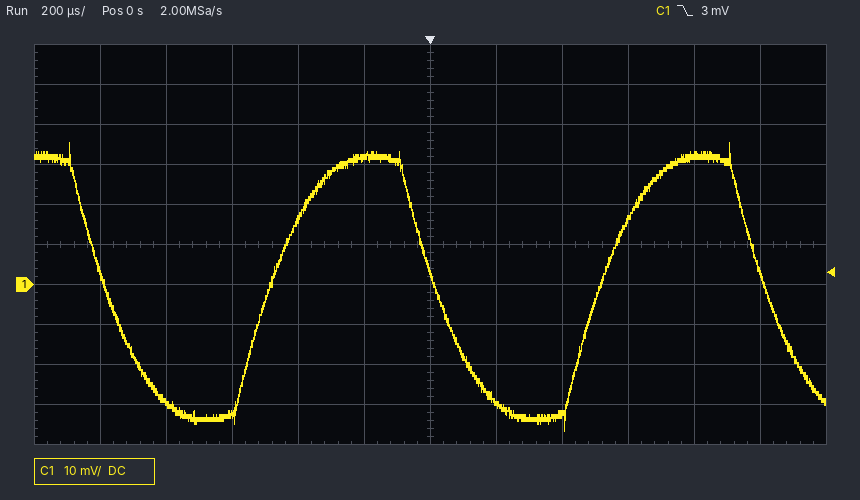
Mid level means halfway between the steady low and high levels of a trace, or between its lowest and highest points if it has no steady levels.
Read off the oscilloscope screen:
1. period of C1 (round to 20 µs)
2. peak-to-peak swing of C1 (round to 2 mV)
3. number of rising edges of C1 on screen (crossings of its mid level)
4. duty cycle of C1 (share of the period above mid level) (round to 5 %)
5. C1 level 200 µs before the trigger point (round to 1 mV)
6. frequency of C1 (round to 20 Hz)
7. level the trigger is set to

1.00 ms
72 mV
2
50 %
32 mV
1.00 kHz
3 mV
